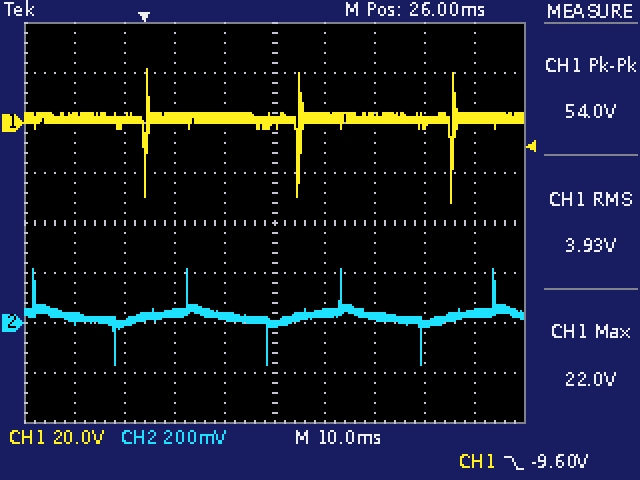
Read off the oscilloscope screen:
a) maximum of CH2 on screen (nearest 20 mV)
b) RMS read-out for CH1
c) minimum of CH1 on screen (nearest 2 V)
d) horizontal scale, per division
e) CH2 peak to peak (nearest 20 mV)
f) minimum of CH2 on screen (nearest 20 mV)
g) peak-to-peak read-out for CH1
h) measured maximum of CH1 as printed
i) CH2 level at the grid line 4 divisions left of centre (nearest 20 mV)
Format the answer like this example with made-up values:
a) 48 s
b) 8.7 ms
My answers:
a) 220 mV
b) 3.93 V
c) -32 V
d) 10 ms
e) 380 mV
f) -160 mV
g) 54.0 V
h) 22.0 V
i) 20 mV
